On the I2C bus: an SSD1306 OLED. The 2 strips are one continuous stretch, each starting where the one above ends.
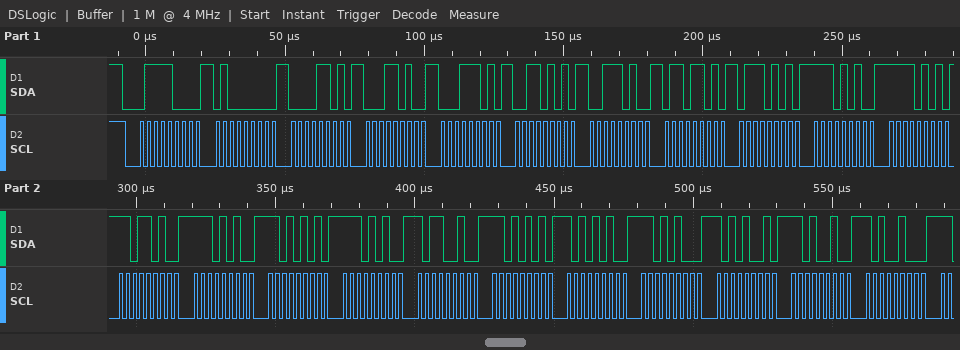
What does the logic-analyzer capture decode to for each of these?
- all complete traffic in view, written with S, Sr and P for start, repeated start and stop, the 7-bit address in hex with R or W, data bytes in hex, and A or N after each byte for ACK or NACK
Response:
S 3CW A 40 A 0D A 1A A 1D A 35 A 3A A 6D A 75 A EA A F5 A DA A EA A D5 A EA A B2 A D5 A AA A D4 A A9 A D2 A A4 A
